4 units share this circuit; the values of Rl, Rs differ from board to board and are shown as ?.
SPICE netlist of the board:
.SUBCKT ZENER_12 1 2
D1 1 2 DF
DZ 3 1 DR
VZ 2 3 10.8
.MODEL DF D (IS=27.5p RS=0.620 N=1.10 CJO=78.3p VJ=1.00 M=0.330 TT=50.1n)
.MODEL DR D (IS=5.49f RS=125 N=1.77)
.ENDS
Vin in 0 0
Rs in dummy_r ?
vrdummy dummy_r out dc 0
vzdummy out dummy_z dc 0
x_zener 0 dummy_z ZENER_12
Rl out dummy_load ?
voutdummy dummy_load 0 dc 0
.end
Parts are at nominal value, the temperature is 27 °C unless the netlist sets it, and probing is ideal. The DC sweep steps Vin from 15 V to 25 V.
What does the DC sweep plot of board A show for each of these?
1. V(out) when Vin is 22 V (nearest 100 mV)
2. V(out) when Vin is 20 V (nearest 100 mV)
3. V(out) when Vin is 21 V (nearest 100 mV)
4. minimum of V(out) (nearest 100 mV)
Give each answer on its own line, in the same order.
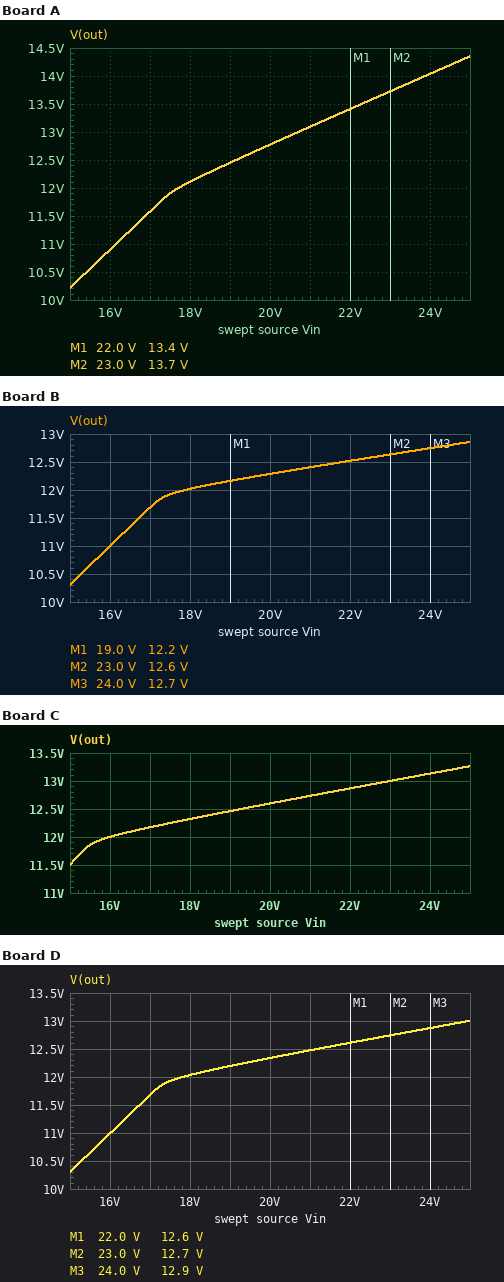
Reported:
13.4 V
12.8 V
13.1 V
10.2 V
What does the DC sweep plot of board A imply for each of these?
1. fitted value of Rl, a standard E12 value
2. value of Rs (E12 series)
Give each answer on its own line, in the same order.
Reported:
470 Ω
220 Ω
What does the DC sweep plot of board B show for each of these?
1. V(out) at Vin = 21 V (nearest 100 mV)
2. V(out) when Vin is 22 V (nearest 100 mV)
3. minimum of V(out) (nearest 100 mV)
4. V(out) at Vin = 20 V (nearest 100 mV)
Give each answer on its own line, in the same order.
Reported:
12.4 V
12.5 V
10.3 V
12.3 V
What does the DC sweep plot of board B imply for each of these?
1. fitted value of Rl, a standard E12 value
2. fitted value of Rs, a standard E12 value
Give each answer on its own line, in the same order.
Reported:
2.2 kΩ
1 kΩ
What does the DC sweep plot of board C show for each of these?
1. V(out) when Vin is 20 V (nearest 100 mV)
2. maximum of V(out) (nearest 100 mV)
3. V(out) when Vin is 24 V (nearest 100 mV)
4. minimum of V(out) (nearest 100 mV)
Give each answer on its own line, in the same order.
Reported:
12.6 V
13.3 V
13.1 V
11.5 V
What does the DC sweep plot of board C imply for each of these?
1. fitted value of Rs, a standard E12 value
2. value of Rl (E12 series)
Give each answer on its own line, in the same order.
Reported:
820 Ω
2.7 kΩ
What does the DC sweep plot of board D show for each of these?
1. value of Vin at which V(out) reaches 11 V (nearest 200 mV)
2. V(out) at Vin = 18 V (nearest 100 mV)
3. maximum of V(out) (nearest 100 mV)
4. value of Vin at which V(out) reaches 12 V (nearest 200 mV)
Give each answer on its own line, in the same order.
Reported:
16.0 V
12.0 V
13.0 V
17.8 V
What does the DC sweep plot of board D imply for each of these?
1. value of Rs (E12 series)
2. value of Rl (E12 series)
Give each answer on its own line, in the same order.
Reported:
820 Ω
1.8 kΩ
